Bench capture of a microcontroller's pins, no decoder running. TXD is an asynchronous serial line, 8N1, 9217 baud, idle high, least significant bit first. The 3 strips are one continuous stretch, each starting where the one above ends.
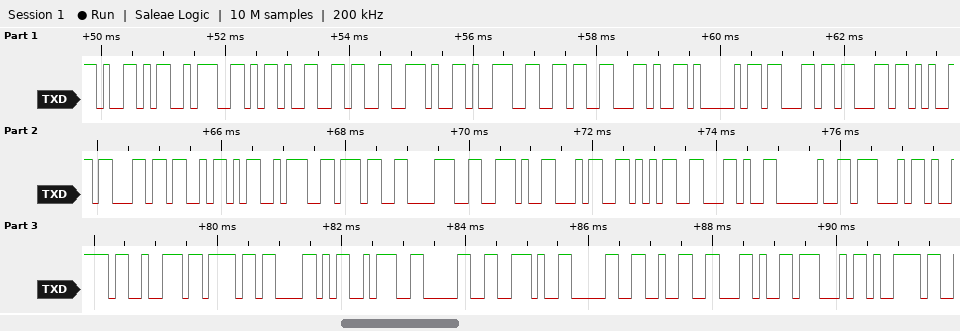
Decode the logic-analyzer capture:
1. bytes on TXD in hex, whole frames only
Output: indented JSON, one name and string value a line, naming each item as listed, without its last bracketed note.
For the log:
{
  "bytes on TXD in hex, whole frames only": "59 3A 2D 36 2E 39 36 2C 41 63 63 65 6C 5A 3A 37 38 2E 34 35 2C 20 47 79 72 6F 58 3A 30 2E 30 32 2C 47 79"
}
